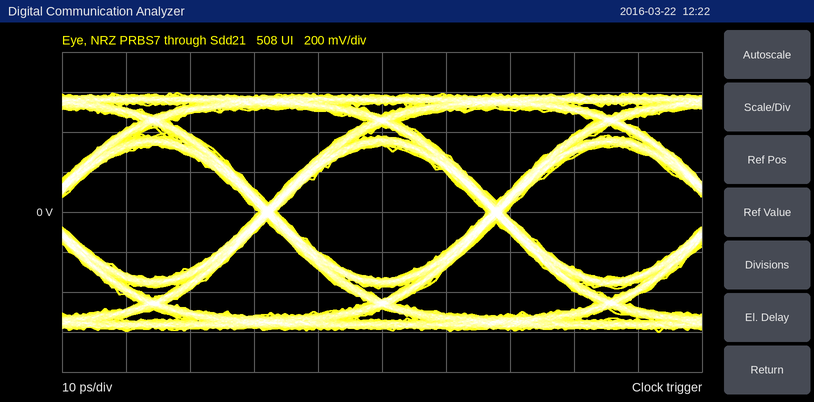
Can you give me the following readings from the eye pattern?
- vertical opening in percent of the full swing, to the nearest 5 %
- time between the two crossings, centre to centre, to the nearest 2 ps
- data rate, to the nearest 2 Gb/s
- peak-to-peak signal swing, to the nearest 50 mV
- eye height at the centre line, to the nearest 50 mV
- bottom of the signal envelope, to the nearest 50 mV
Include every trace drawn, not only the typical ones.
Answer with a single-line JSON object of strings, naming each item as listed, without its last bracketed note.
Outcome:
{"vertical opening in percent of the full swing, to the nearest 5 %": "55 %", "time between the two crossings, centre to centre, to the nearest 2 ps": "36 ps", "data rate, to the nearest 2 Gb/s": "28 Gb/s", "peak-to-peak signal swing, to the nearest 50 mV": "1.20 V", "eye height at the centre line, to the nearest 50 mV": "650 mV", "bottom of the signal envelope, to the nearest 50 mV": "-600 mV"}
